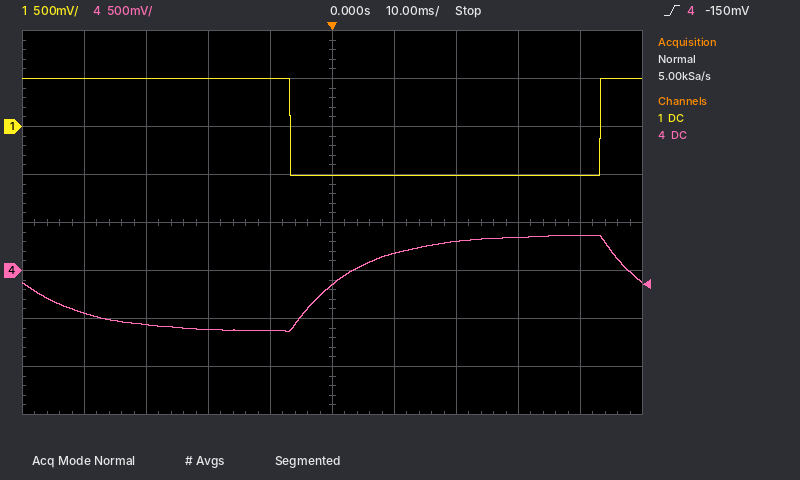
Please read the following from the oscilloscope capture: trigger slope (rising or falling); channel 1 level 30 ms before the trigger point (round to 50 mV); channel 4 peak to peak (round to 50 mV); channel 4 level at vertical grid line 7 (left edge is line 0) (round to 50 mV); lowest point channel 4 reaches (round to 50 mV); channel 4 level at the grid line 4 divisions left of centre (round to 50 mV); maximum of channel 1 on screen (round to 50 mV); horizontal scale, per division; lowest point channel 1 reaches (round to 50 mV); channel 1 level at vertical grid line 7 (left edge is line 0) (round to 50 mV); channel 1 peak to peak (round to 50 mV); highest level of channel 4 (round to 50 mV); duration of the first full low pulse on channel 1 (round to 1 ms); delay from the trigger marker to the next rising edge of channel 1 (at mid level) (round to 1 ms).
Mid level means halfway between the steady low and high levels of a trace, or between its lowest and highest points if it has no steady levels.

rising
500 mV
1.00 V
300 mV
-650 mV
-450 mV
500 mV
10 ms
-500 mV
-500 mV
1.00 V
350 mV
50 ms
43 ms
